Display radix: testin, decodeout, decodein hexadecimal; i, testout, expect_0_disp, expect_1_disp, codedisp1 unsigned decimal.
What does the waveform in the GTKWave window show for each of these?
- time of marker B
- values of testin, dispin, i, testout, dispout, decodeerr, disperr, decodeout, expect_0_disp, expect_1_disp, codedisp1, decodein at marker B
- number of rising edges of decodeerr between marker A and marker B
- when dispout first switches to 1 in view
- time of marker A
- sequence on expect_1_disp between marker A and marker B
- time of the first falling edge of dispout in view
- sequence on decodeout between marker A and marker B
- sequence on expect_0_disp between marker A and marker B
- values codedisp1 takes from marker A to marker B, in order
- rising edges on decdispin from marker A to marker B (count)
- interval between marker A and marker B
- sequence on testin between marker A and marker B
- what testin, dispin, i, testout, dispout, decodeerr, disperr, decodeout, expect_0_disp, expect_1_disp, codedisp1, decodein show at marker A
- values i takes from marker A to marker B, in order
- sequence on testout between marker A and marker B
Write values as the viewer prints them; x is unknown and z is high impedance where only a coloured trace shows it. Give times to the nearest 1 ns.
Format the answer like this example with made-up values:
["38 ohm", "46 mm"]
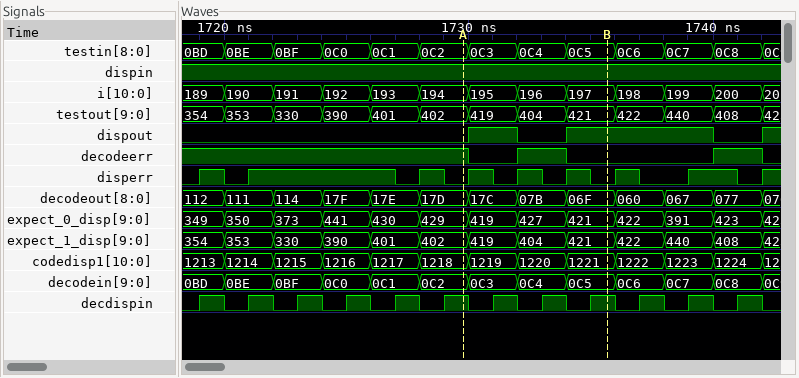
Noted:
["1736 ns", "testin=0C5, dispin=1, i=197, testout=421, dispout=1, decodeerr=0, disperr=0, decodeout=06F, expect_0_disp=421, expect_1_disp=421, codedisp1=1221, decodein=0C5", "1", "1730 ns", "1730 ns", "402, 419, 404, 421", "1732 ns", "17D, 17C, 07B, 06F", "429, 419, 427, 421", "1218, 1219, 1220, 1221", "3", "6 ns", "0C2, 0C3, 0C4, 0C5", "testin=0C2, dispin=1, i=194, testout=402, dispout=0, decodeerr=1, disperr=0, decodeout=17D, expect_0_disp=429, expect_1_disp=402, codedisp1=1218, decodein=0C2", "194, 195, 196, 197", "402, 419, 404, 421"]
